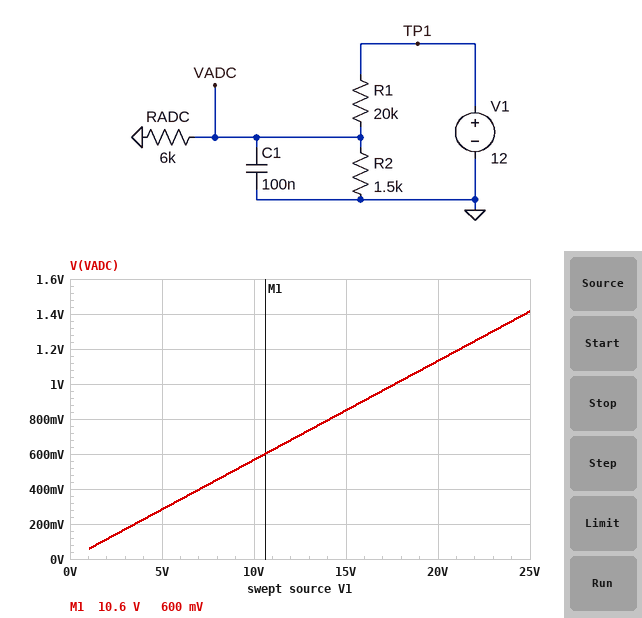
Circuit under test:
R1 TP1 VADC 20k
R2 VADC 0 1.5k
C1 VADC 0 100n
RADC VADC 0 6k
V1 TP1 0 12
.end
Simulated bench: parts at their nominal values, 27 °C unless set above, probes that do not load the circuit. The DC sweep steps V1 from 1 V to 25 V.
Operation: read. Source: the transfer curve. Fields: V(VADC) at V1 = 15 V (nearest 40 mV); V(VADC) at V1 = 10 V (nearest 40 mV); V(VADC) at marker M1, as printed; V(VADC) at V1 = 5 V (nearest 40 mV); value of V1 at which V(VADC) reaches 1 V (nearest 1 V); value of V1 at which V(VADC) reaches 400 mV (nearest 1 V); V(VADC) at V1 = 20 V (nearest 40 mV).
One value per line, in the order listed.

840 mV
560 mV
600 mV
280 mV
18 V
7 V
1.12 V
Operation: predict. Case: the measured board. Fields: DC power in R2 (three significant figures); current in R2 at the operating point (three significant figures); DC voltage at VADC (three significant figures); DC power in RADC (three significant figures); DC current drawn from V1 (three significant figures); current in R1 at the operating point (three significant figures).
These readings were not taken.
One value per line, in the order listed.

308 µW
453 µA
679 mV
76.9 µW
566 µA
566 µA
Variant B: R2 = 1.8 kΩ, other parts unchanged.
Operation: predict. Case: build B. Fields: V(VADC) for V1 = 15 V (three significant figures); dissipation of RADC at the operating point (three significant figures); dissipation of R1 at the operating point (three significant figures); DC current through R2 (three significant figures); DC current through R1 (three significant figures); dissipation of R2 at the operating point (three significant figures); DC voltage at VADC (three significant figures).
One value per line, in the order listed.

971 mV
101 µW
6.30 mW
432 µA
561 µA
335 µW
777 mV
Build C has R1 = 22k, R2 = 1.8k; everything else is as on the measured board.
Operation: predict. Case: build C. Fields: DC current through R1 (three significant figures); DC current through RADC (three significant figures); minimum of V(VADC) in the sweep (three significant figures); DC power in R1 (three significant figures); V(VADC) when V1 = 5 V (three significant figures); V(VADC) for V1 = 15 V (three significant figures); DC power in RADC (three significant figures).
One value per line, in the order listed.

513 µA
118 µA
59.2 mV
5.79 mW
296 mV
888 mV
84.1 µW
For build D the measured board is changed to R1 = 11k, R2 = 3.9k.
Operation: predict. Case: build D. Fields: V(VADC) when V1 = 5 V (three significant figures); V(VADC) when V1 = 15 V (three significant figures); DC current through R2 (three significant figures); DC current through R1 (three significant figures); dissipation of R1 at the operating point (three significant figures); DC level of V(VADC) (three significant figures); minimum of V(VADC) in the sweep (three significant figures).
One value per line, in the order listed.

884 mV
2.65 V
544 µA
898 µA
8.87 mW
2.12 V
177 mV
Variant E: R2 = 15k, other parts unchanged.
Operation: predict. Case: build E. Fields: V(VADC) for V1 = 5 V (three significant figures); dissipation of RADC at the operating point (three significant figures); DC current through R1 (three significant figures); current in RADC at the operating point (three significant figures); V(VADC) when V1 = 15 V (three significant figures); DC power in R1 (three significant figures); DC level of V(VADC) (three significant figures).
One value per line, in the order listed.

882 mV
747 µW
494 µA
353 µA
2.65 V
4.88 mW
2.12 V
